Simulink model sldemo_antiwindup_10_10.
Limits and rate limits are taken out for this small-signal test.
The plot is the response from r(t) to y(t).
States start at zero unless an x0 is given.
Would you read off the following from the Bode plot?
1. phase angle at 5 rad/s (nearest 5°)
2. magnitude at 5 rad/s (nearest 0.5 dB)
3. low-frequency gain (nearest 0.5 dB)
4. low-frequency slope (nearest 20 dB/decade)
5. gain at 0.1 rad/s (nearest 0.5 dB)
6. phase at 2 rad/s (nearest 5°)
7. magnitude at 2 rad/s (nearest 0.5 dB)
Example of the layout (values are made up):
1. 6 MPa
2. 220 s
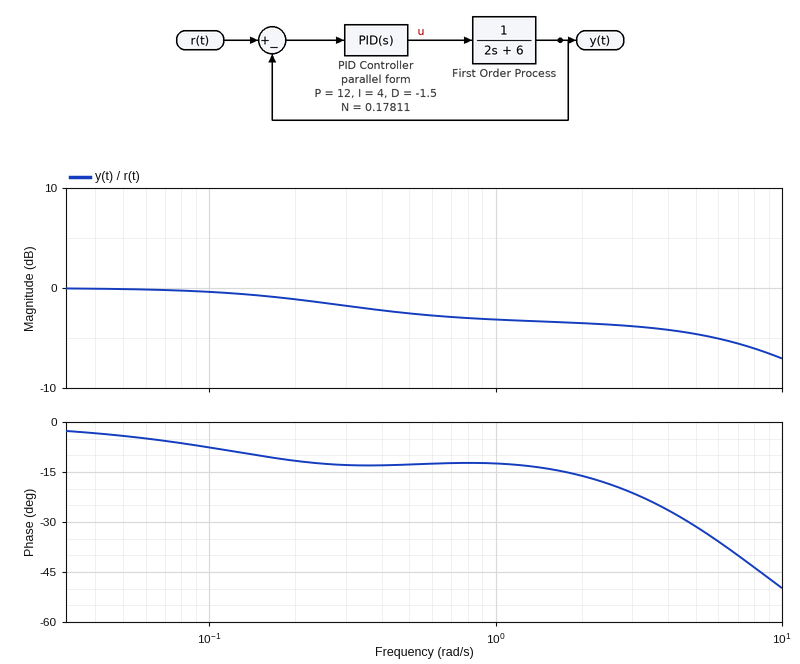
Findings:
1. -30°
2. -4.5 dB
3. 0.0 dB
4. 0 dB/decade
5. -0.5 dB
6. -15°
7. -3.5 dB
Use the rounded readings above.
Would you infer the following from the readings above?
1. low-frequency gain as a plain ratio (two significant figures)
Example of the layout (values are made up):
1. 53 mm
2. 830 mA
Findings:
1. 1.0
